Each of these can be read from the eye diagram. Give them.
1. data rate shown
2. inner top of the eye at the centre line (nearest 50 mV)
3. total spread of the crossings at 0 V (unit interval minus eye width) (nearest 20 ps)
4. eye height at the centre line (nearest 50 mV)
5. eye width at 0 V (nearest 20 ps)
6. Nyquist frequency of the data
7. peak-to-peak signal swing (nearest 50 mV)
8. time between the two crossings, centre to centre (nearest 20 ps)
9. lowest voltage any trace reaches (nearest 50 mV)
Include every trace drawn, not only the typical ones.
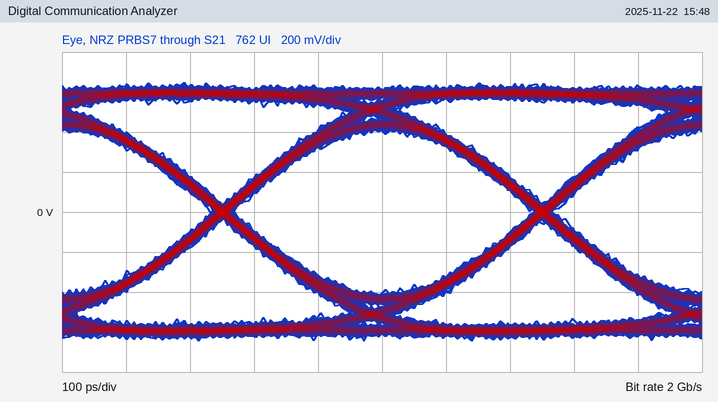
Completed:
2 Gb/s
400 mV
40 ps
800 mV
460 ps
1 GHz
1.30 V
500 ps
-650 mV
